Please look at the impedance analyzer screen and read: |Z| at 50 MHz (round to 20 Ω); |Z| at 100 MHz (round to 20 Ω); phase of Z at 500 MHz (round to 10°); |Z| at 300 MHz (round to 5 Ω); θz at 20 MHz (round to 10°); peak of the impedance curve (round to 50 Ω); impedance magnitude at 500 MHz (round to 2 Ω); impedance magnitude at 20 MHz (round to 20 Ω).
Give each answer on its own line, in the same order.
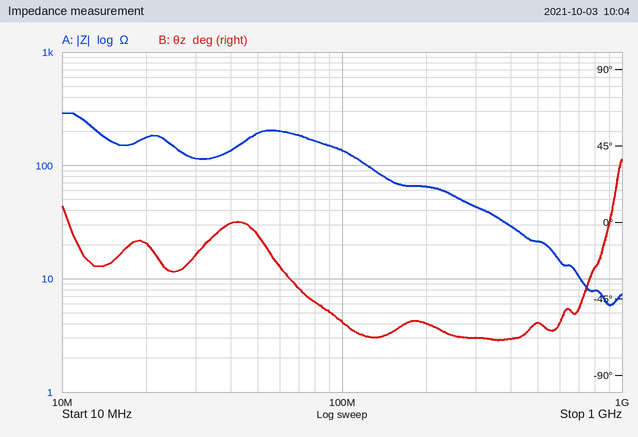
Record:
200 Ω
140 Ω
-60°
45 Ω
-10°
300 Ω
22 Ω
180 Ω
